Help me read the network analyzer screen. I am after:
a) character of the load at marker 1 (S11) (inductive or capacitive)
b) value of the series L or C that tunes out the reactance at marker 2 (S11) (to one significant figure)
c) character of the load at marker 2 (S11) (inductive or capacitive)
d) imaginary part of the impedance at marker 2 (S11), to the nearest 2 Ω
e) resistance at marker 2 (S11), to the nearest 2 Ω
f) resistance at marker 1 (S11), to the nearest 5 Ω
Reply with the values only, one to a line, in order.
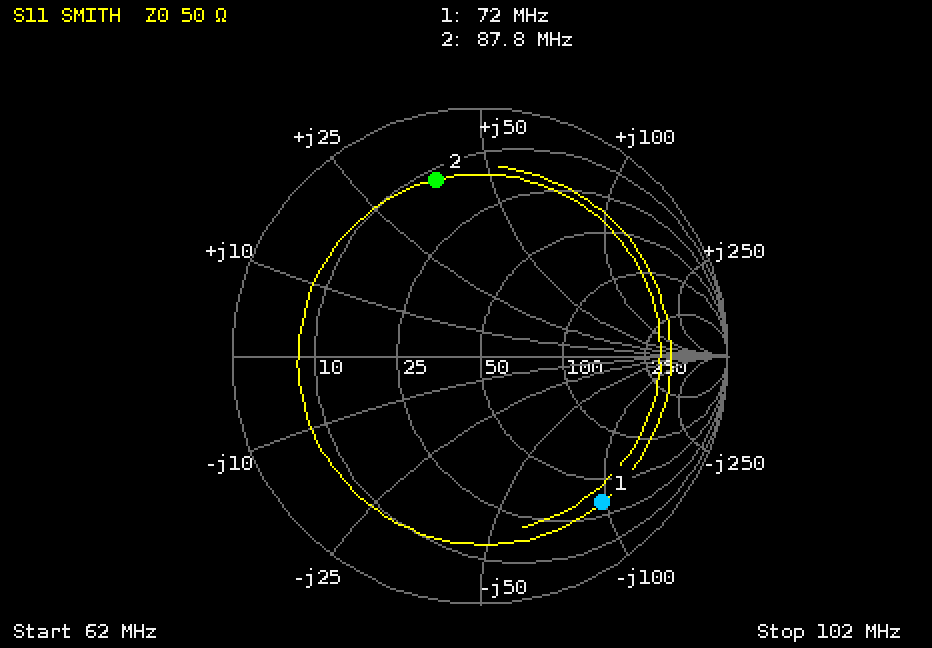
capacitive
50 pF
inductive
+38 Ω
12 Ω
35 Ω
